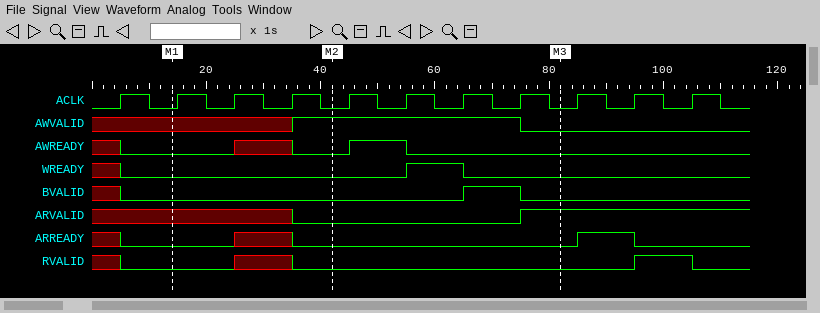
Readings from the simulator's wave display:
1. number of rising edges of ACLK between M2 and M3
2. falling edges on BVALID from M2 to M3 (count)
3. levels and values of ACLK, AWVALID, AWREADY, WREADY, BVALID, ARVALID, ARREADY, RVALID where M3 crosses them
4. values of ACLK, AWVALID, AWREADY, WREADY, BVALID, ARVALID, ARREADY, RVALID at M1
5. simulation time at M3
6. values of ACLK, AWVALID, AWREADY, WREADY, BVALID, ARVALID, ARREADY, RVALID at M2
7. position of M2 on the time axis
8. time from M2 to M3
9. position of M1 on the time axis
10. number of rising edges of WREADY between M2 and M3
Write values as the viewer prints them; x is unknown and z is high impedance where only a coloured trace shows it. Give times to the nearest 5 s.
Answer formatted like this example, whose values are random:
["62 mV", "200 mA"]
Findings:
["4", "1", "ACLK=0, AWVALID=0, AWREADY=0, WREADY=0, BVALID=0, ARVALID=1, ARREADY=0, RVALID=0", "ACLK=0, AWVALID=x, AWREADY=0, WREADY=0, BVALID=0, ARVALID=x, ARREADY=0, RVALID=0", "80 s", "ACLK=0, AWVALID=1, AWREADY=0, WREADY=0, BVALID=0, ARVALID=0, ARREADY=0, RVALID=0", "40 s", "40 s", "15 s", "1"]
